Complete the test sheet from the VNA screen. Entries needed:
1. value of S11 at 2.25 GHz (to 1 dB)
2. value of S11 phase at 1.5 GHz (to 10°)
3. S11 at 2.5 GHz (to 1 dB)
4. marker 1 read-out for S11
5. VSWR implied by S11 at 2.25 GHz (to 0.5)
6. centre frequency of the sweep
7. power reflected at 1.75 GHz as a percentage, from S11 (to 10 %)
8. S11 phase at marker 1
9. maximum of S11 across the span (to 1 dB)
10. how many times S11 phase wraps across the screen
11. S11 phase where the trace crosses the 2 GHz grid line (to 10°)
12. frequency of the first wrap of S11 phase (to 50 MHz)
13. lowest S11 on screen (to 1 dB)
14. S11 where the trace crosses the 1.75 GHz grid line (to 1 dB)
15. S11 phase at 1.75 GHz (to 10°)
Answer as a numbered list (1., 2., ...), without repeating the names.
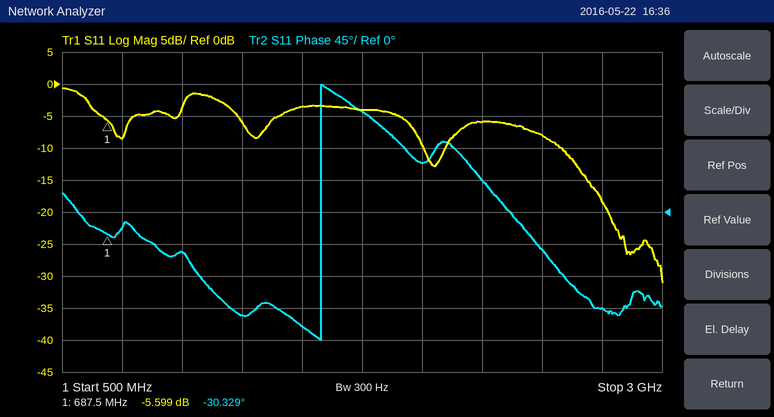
1. -6 dB
2. -160°
3. -8 dB
4. -5.599 dB
5. 3.0
6. 1.75 GHz
7. 40 %
8. -30.329°
9. -1 dB
10. 1
11. 70°
12. 1.60 GHz
13. -31 dB
14. -4 dB
15. 140°
